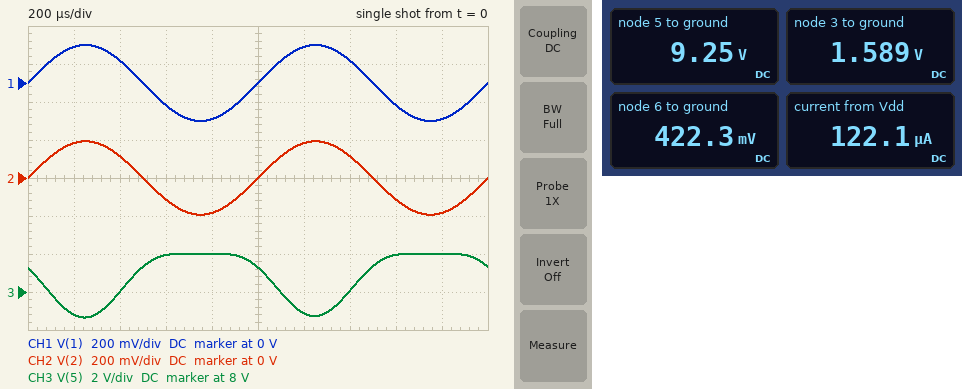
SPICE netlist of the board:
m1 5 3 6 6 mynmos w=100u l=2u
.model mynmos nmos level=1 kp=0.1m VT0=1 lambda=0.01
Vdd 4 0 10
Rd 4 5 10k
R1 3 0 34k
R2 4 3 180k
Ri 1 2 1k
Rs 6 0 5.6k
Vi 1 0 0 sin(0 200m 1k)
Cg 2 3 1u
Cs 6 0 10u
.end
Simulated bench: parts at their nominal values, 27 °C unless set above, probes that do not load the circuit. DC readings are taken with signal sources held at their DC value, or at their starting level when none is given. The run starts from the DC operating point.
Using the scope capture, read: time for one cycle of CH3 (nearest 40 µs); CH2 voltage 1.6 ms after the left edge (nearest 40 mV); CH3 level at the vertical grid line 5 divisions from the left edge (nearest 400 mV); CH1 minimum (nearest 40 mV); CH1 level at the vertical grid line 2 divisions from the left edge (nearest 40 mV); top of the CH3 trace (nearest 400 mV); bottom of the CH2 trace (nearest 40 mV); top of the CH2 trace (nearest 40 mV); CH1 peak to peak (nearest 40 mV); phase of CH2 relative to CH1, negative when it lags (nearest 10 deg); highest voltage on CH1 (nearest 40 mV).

1.00 ms
-120 mV
9.2 V
-200 mV
120 mV
10.0 V
-200 mV
200 mV
400 mV
0 deg
200 mV
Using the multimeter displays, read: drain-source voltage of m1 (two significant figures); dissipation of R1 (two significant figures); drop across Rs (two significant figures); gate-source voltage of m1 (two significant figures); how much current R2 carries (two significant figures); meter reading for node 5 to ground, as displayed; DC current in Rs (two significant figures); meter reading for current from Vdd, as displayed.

8.8 V
74 µW
420 mV
1.2 V
47 µA
9.25 V
75 µA
122.1 µA
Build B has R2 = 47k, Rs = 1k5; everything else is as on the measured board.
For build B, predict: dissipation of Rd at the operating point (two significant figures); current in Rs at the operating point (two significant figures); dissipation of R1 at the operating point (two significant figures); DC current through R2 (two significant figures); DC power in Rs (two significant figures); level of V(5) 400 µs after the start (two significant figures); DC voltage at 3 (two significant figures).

7.4 mW
860 µA
520 µW
120 µA
1.1 mW
1.4 V
4.2 V
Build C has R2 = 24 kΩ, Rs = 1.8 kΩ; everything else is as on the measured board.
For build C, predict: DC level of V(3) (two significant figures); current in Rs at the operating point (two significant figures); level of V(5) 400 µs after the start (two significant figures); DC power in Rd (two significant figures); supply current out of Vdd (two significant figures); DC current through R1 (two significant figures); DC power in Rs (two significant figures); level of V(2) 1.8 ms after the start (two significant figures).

5.9 V
840 µA
1.6 V
7.1 mW
1.0 mA
170 µA
1.3 mW
-180 mV
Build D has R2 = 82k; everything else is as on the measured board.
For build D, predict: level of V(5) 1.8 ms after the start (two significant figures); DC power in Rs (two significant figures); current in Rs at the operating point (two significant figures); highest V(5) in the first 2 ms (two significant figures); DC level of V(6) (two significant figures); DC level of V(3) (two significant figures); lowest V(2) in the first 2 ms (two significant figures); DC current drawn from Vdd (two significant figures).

9.5 V
460 µW
290 µA
9.6 V
1.6 V
2.9 V
-190 mV
370 µA
